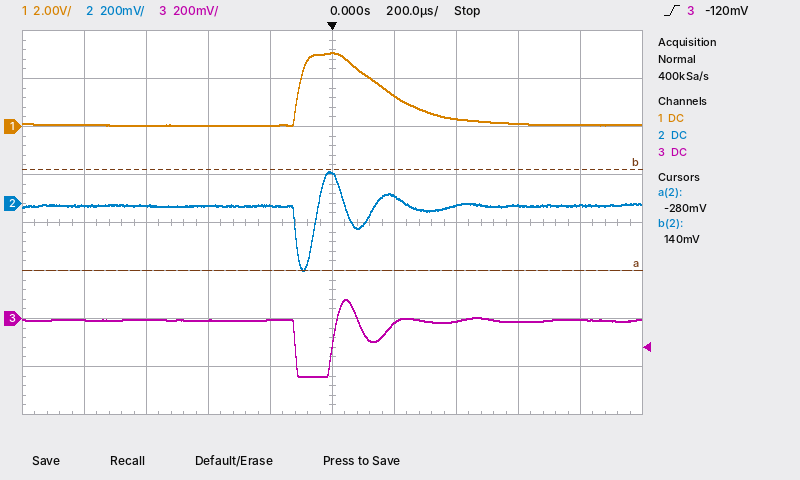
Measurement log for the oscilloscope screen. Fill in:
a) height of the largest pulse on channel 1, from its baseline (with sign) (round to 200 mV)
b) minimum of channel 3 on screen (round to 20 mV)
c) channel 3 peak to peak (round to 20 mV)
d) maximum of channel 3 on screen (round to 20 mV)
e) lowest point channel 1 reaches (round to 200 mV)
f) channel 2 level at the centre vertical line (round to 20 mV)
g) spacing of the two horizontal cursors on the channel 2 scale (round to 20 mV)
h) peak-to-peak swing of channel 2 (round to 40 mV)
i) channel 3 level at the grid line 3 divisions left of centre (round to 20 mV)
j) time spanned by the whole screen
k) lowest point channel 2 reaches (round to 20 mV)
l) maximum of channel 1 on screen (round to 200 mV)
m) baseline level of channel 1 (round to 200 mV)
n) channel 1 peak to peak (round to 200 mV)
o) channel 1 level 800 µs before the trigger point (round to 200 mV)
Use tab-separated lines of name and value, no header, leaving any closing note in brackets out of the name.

height of the largest pulse on channel 1, from its baseline (with sign)	+3.0 V
minimum of channel 3 on screen	-240 mV
channel 3 peak to peak	320 mV
maximum of channel 3 on screen	80 mV
lowest point channel 1 reaches	0.0 V
channel 2 level at the centre vertical line	120 mV
spacing of the two horizontal cursors on the channel 2 scale	420 mV
peak-to-peak swing of channel 2	400 mV
channel 3 level at the grid line 3 divisions left of centre	0 mV
time spanned by the whole screen	2 ms
lowest point channel 2 reaches	-280 mV
maximum of channel 1 on screen	3.0 V
baseline level of channel 1	0.0 V
channel 1 peak to peak	3.0 V
channel 1 level 800 µs before the trigger point	0.0 V
